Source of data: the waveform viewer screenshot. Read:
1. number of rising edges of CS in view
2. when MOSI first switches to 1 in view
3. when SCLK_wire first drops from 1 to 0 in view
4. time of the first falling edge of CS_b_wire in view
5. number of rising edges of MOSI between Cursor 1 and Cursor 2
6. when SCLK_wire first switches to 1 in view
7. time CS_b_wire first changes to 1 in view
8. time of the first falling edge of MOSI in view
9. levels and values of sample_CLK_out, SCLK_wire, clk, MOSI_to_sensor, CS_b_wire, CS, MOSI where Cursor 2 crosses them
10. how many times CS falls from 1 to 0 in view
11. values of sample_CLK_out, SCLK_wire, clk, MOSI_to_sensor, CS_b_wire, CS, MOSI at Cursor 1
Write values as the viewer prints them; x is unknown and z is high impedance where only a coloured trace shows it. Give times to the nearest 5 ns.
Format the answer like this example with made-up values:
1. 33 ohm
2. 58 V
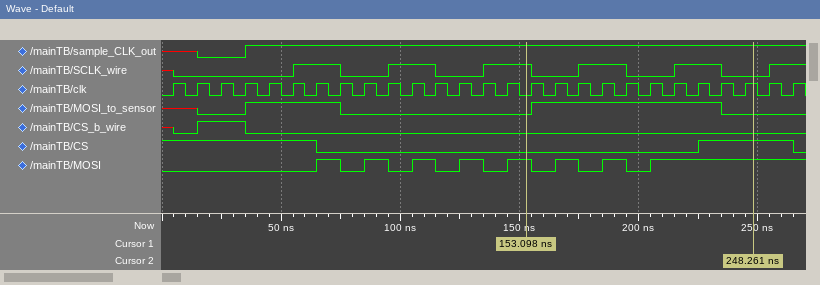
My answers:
1. 1
2. 65 ns
3. 75 ns
4. 35 ns
5. 3
6. 55 ns
7. 15 ns
8. 75 ns
9. sample_CLK_out=1, SCLK_wire=0, clk=1, MOSI_to_sensor=0, CS_b_wire=0, CS=1, MOSI=1
10. 2
11. sample_CLK_out=1, SCLK_wire=1, clk=0, MOSI_to_sensor=0, CS_b_wire=0, CS=0, MOSI=1
